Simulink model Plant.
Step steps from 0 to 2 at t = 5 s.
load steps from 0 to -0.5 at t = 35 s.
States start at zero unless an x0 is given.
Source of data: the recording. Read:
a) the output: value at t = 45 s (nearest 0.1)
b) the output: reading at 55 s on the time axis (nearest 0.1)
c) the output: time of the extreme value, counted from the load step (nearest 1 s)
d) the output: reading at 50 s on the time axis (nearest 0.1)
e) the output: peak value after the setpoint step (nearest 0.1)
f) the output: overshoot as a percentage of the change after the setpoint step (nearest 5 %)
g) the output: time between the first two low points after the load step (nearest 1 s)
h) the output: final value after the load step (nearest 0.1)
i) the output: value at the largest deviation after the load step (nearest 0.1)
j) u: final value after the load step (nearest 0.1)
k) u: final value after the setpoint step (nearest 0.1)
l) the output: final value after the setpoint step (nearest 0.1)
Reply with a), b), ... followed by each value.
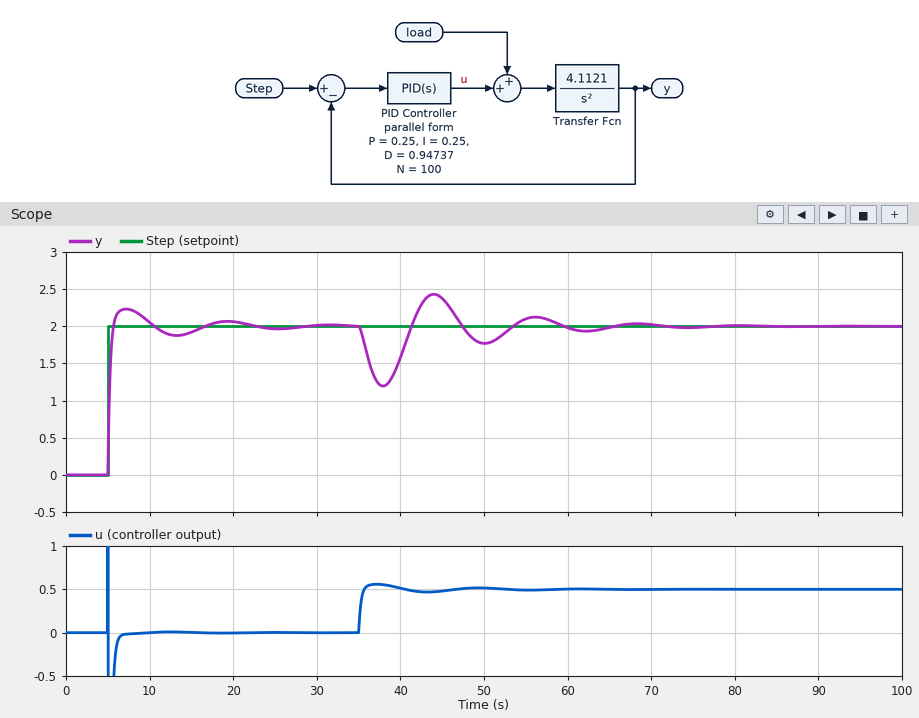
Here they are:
a) 2.4
b) 2.1
c) 3 s
d) 1.8
e) 2.2
f) 10 %
g) 12 s
h) 2.0
i) 1.2
j) 0.5
k) 0.0
l) 2.0
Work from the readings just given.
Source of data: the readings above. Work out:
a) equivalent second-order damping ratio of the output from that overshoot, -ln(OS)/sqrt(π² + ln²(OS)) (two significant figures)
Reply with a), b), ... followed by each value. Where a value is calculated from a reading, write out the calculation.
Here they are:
a) ln(0.1) = -2.303; 2.303 / sqrt(9.870 + 5.302) = 0.59
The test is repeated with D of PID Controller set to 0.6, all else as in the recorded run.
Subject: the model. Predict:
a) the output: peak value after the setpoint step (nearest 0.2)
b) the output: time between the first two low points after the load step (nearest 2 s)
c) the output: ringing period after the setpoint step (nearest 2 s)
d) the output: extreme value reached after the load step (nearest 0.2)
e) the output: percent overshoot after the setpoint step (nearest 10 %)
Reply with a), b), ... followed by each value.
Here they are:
a) 2.4
b) 10 s
c) 10 s
d) 1.0
e) 20 %
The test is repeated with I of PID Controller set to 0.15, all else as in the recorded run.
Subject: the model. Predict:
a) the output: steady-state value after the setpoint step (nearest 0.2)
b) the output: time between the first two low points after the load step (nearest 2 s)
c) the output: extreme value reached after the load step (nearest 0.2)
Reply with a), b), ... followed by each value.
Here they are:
a) 2.0
b) 16 s
c) 1.0
